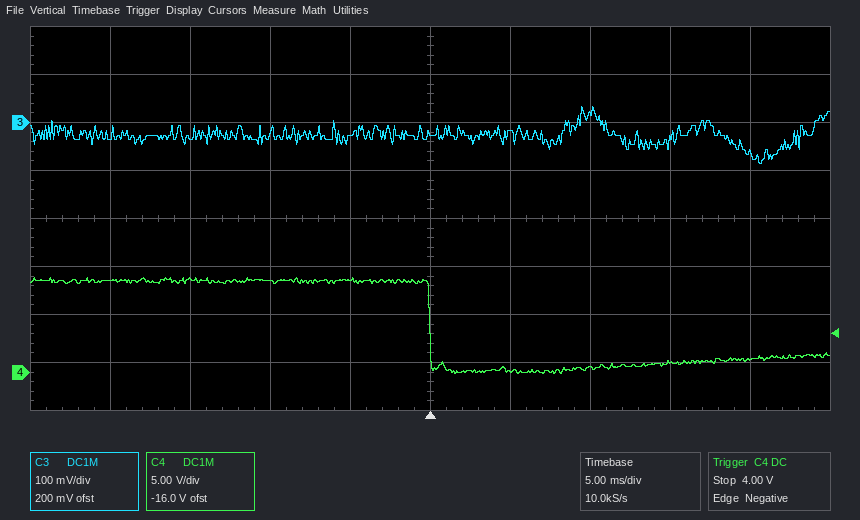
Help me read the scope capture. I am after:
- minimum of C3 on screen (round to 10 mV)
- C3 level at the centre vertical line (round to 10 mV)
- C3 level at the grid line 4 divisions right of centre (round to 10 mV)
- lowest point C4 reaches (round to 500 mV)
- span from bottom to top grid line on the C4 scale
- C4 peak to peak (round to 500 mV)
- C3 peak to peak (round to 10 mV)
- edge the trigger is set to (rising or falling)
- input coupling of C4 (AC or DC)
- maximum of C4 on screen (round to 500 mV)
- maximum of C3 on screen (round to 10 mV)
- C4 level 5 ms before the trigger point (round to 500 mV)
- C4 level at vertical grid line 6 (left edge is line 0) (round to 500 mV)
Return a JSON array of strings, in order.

["-90 mV", "-30 mV", "-70 mV", "0.0 V", "40 V", "10.0 V", "120 mV", "falling", "DC", "10.0 V", "30 mV", "9.5 V", "0.0 V"]
